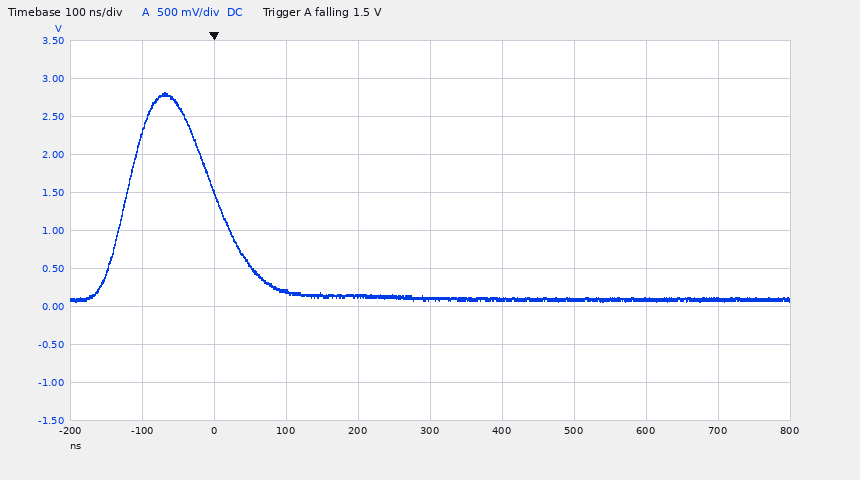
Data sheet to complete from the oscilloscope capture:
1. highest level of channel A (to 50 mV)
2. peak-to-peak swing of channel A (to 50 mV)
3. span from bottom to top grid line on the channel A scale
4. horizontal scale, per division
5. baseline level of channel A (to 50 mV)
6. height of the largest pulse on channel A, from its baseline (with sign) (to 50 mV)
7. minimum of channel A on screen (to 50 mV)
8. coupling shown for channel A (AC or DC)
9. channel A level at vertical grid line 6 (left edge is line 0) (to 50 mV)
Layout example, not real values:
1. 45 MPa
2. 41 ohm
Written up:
1. 2.80 V
2. 2.75 V
3. 5 V
4. 100 ns
5. 100 mV
6. +2.70 V
7. 50 mV
8. DC
9. 100 mV
